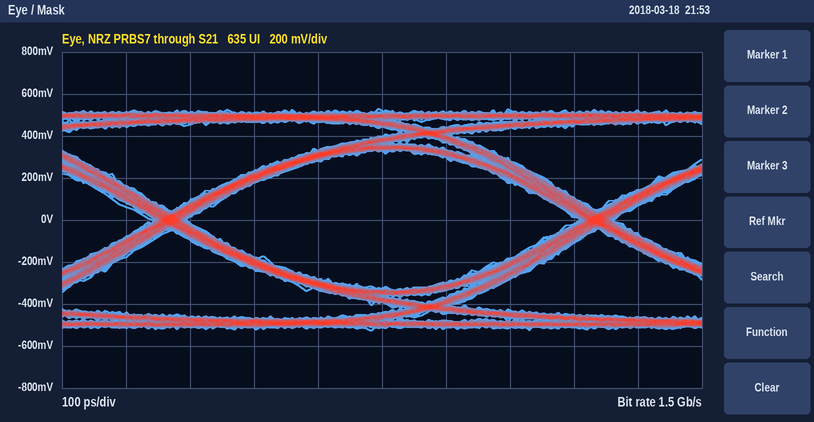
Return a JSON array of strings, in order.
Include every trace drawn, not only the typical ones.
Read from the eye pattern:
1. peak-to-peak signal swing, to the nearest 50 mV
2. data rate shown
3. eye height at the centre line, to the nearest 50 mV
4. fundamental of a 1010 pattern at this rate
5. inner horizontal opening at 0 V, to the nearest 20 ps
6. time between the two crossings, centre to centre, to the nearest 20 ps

["1.05 V", "1.5 Gb/s", "650 mV", "750 MHz", "620 ps", "660 ps"]
